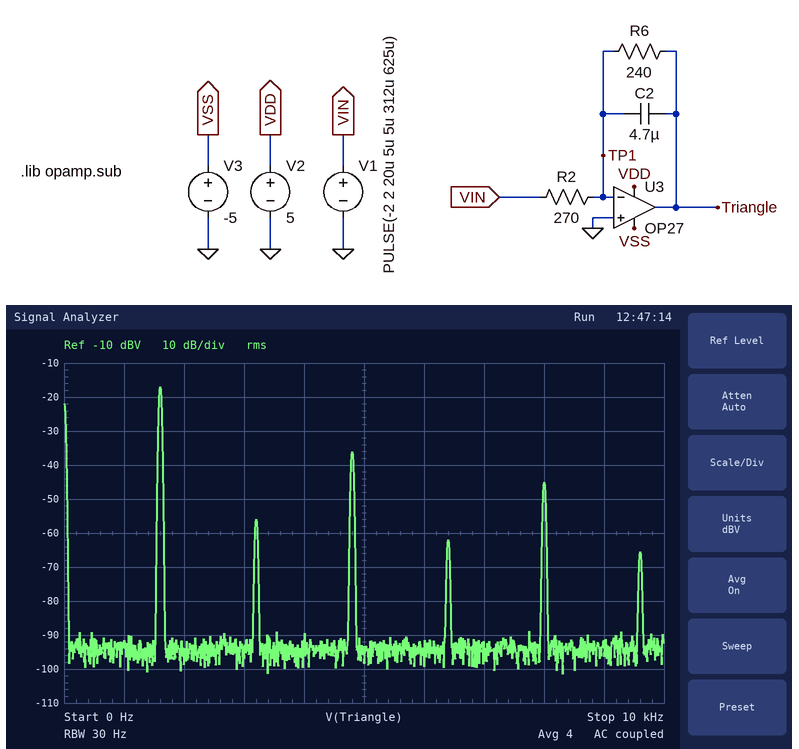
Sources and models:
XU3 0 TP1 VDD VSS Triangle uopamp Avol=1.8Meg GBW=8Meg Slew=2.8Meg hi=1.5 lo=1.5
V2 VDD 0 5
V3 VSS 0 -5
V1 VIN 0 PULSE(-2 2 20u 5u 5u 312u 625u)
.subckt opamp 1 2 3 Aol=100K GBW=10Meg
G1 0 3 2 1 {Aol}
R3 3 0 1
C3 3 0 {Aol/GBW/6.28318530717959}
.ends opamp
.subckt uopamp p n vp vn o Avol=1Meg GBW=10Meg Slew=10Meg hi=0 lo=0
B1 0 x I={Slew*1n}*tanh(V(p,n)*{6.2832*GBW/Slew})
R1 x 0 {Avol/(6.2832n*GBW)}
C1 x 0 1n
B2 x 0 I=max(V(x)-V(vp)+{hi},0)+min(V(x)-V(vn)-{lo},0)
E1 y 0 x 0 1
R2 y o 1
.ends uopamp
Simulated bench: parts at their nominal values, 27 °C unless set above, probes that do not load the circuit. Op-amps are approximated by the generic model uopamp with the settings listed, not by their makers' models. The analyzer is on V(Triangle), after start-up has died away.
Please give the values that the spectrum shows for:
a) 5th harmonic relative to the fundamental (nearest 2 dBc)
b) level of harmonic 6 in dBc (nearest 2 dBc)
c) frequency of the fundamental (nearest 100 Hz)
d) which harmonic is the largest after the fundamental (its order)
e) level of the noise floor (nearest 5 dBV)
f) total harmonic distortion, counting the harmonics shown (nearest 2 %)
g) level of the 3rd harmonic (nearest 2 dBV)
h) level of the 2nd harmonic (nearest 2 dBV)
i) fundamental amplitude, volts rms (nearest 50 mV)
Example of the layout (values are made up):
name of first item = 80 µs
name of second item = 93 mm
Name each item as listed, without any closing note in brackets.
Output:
5th harmonic relative to the fundamental = -28 dBc
level of harmonic 6 in dBc = -48 dBc
frequency of the fundamental = 1.6 kHz
which harmonic is the largest after the fundamental = 3
level of the noise floor = -95 dBV
total harmonic distortion, counting the harmonics shown = 12 %
level of the 3rd harmonic = -36 dBV
level of the 2nd harmonic = -56 dBV
fundamental amplitude, volts rms = 150 mV
